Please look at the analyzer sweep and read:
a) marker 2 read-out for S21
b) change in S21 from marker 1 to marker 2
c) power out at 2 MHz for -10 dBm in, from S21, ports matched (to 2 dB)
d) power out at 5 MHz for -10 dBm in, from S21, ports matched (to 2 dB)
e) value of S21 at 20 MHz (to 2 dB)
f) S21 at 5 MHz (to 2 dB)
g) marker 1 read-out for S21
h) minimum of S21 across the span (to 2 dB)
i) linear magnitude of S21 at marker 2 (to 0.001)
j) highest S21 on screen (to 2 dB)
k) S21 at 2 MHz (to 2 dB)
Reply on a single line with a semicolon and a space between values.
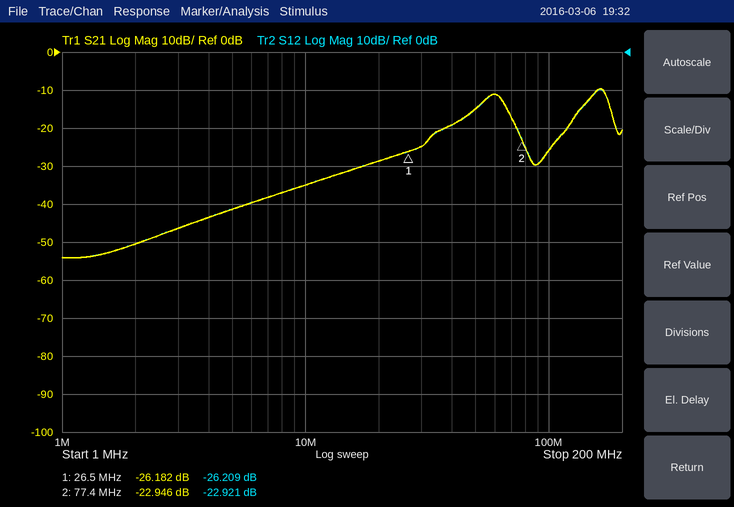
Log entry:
-22.946 dB; 3.236 dB; -60 dBm; -52 dBm; -28 dB; -42 dB; -26.182 dB; -54 dB; 0.071; -10 dB; -50 dB
